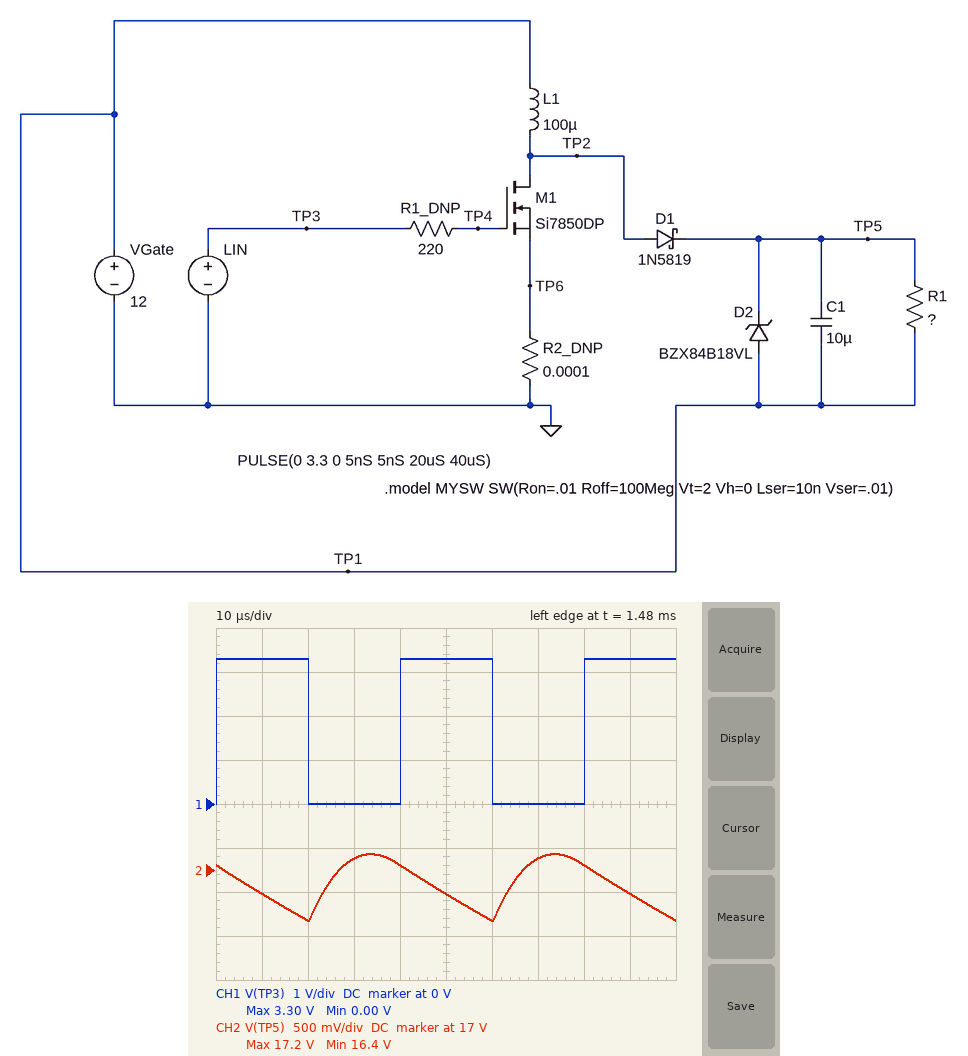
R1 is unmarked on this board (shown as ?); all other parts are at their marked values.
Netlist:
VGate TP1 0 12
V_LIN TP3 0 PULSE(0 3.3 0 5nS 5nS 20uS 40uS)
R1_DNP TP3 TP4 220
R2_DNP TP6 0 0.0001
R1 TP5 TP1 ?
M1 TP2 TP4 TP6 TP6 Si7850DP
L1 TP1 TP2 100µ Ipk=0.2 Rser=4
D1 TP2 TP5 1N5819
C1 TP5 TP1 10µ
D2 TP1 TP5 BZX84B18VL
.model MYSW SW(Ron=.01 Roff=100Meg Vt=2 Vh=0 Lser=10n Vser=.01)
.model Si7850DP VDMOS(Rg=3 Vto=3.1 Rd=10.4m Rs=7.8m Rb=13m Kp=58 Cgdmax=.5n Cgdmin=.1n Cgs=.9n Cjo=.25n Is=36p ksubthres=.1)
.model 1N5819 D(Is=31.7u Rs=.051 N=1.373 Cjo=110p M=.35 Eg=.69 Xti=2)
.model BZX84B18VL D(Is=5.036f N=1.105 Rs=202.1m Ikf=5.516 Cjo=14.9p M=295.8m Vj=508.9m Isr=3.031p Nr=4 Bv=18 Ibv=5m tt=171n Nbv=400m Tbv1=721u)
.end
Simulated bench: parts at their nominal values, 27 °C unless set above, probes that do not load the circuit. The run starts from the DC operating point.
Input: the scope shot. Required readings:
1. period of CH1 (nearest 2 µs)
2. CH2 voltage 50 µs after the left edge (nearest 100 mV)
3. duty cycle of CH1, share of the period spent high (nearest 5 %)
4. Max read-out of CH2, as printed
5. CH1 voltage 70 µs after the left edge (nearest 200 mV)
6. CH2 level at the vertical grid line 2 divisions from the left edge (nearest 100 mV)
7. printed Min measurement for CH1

40 µs
16.7 V
50 %
17.2 V
0 V
16.4 V
0.00 V
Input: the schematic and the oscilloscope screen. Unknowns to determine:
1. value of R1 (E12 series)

15 Ω
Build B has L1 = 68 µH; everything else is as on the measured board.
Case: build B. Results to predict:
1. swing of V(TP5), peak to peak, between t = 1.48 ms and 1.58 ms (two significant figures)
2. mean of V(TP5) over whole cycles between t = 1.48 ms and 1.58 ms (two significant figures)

780 mV
16 V
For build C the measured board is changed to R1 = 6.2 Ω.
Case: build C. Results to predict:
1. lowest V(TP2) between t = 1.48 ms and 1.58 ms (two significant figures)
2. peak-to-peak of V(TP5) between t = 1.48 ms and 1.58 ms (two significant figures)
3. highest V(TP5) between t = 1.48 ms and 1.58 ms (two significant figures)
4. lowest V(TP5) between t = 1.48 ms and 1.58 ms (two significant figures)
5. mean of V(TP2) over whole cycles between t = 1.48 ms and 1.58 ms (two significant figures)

81 mV
840 mV
15 V
14 V
8.5 V
